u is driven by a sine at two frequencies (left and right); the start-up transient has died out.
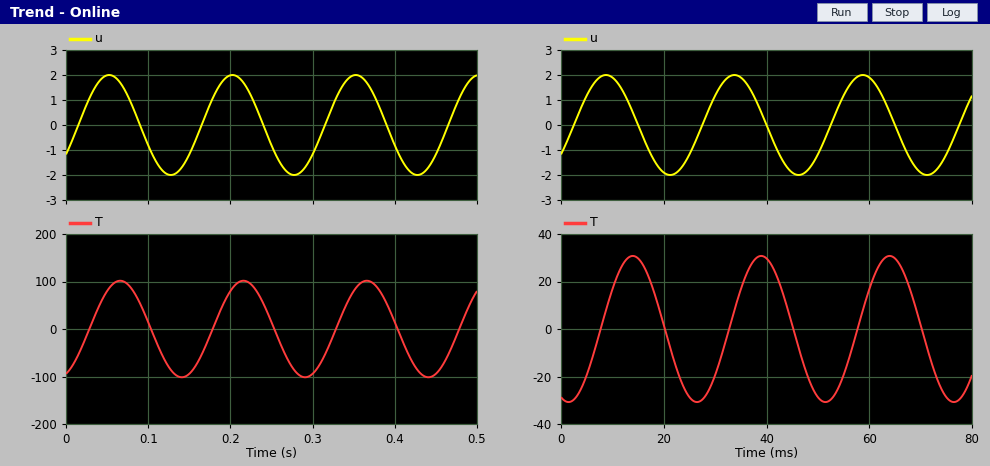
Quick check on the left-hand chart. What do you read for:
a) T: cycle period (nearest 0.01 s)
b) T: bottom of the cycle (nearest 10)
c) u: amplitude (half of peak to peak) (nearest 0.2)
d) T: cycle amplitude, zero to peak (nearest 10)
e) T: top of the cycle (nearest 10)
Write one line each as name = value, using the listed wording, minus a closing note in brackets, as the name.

T: cycle period = 0.15 s
T: bottom of the cycle = -100
u: amplitude (half of peak to peak) = 2.0
T: cycle amplitude, zero to peak = 100
T: top of the cycle = 100
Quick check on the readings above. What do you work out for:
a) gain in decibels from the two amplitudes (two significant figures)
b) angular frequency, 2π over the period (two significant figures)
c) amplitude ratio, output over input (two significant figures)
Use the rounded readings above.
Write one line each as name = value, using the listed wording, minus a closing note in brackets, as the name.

gain in decibels from the two amplitudes = 34 dB
angular frequency, 2π over the period = 42 rad/s
amplitude ratio, output over input = 50
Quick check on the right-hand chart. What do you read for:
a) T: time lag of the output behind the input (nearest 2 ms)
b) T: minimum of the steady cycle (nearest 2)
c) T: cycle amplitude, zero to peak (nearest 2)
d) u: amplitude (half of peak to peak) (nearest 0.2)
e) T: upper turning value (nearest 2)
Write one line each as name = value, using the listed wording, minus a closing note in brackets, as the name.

T: time lag of the output behind the input = 6 ms
T: minimum of the steady cycle = -30
T: cycle amplitude, zero to peak = 30
u: amplitude (half of peak to peak) = 2.0
T: upper turning value = 30
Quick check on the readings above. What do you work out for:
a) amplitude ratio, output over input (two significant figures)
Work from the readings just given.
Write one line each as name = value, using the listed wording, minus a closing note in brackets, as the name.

amplitude ratio, output over input = 15
